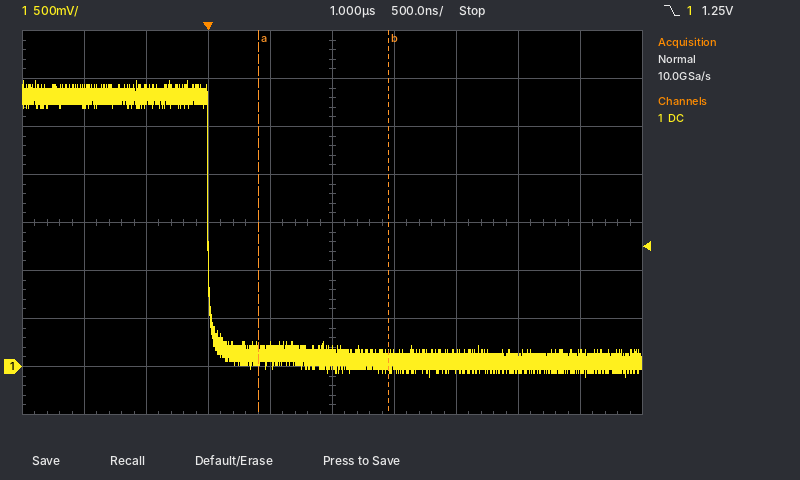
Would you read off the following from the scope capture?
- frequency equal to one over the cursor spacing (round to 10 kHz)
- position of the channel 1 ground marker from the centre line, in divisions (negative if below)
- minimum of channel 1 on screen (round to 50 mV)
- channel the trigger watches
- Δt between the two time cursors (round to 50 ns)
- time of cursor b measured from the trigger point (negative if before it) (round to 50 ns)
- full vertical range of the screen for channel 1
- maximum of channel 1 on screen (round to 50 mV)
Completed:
950 kHz
-3.0 div
-100 mV
channel 1
1.05 µs
+1.45 µs
4 V
3.00 V
